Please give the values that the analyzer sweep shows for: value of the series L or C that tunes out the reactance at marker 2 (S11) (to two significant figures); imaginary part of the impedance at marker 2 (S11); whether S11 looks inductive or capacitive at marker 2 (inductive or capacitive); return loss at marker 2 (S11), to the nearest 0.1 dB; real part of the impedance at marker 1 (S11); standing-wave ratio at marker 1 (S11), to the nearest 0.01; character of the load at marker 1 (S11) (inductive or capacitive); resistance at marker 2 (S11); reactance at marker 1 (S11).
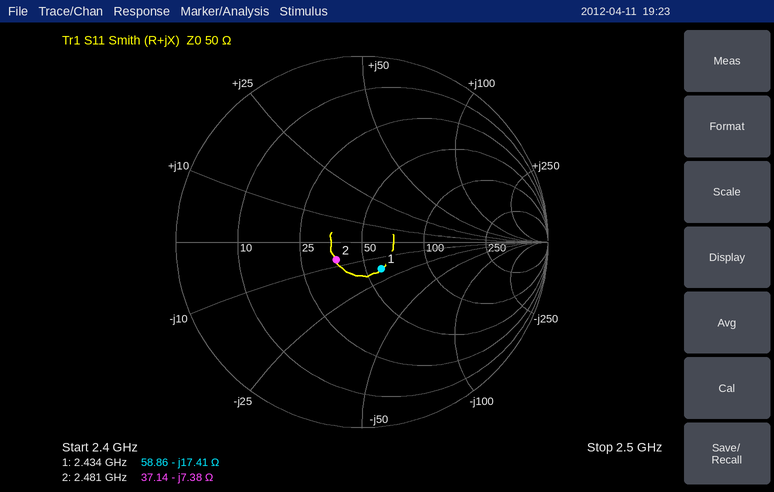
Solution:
470 pH
-7.38 Ω
capacitive
15.4 dB
58.86 Ω
1.43
capacitive
37.14 Ω
-17.41 Ω
